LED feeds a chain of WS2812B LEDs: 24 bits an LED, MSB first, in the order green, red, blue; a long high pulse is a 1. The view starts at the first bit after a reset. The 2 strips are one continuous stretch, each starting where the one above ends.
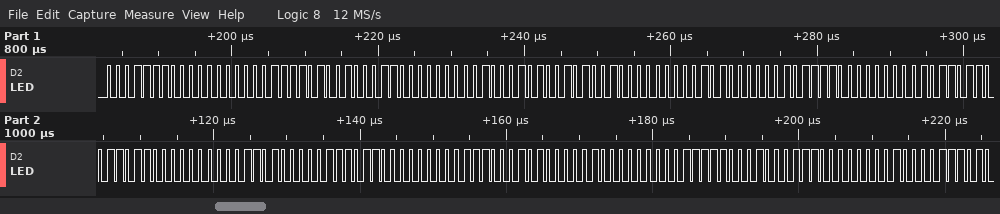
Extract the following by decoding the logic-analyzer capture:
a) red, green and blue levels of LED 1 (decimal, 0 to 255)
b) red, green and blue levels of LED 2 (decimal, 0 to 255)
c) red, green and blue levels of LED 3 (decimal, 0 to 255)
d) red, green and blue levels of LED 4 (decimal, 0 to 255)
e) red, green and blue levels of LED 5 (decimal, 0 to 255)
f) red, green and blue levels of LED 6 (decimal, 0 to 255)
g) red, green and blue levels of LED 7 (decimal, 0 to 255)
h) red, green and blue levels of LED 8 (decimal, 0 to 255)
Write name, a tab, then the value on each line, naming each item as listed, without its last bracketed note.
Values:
red, green and blue levels of LED 1	0, 30, 61
red, green and blue levels of LED 2	0, 35, 69
red, green and blue levels of LED 3	0, 41, 80
red, green and blue levels of LED 4	0, 47, 91
red, green and blue levels of LED 5	0, 54, 104
red, green and blue levels of LED 6	0, 59, 113
red, green and blue levels of LED 7	0, 65, 124
red, green and blue levels of LED 8	0, 71, 135
